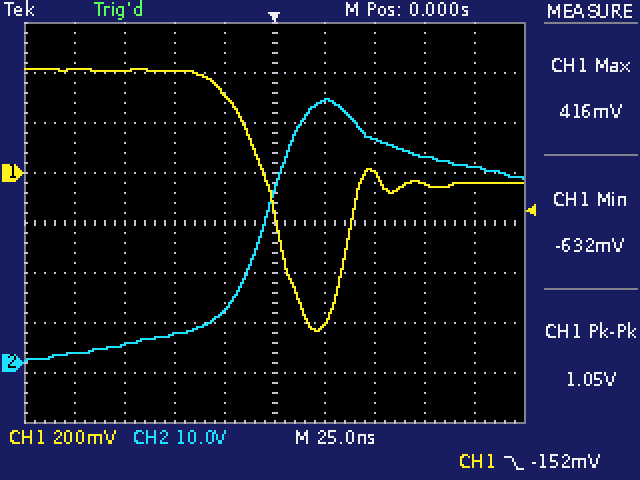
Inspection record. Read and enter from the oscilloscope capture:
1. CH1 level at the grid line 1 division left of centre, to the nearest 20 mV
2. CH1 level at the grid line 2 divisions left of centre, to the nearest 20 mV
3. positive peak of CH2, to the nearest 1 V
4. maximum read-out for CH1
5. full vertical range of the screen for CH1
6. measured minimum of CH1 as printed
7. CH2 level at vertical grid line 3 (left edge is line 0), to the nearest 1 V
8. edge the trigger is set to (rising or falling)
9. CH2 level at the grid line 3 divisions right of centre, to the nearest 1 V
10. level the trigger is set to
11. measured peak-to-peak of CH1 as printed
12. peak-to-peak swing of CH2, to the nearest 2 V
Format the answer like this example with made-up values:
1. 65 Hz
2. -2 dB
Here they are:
1. 320 mV
2. 400 mV
3. 53 V
4. 416 mV
5. 1.6 V
6. -632 mV
7. 6 V
8. falling
9. 41 V
10. -152 mV
11. 1.05 V
12. 52 V
